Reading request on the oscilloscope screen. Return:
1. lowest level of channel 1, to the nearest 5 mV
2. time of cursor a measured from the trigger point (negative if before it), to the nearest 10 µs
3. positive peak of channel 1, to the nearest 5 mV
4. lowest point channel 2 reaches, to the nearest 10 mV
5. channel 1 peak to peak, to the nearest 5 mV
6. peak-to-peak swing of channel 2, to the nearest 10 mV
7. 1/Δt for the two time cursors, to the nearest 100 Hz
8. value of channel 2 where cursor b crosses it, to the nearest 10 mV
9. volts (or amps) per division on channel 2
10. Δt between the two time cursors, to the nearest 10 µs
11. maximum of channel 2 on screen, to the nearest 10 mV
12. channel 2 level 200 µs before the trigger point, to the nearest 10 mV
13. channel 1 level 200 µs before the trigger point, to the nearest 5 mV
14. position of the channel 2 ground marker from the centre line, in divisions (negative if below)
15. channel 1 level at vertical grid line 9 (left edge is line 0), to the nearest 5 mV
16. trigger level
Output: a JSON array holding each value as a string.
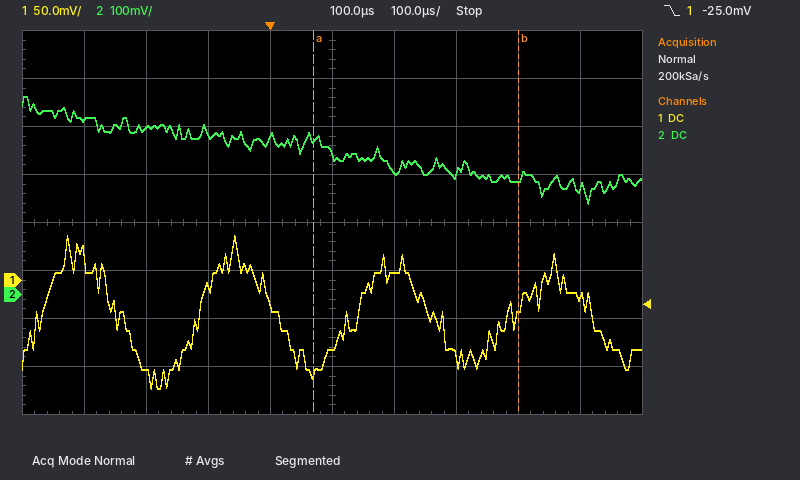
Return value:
["-115 mV", "+70 µs", "45 mV", "190 mV", "160 mV", "220 mV", "3.0 kHz", "240 mV", "100 mV", "330 µs", "410 mV", "350 mV", "-95 mV", "-1.5 div", "-15 mV", "-25.0 mV"]
